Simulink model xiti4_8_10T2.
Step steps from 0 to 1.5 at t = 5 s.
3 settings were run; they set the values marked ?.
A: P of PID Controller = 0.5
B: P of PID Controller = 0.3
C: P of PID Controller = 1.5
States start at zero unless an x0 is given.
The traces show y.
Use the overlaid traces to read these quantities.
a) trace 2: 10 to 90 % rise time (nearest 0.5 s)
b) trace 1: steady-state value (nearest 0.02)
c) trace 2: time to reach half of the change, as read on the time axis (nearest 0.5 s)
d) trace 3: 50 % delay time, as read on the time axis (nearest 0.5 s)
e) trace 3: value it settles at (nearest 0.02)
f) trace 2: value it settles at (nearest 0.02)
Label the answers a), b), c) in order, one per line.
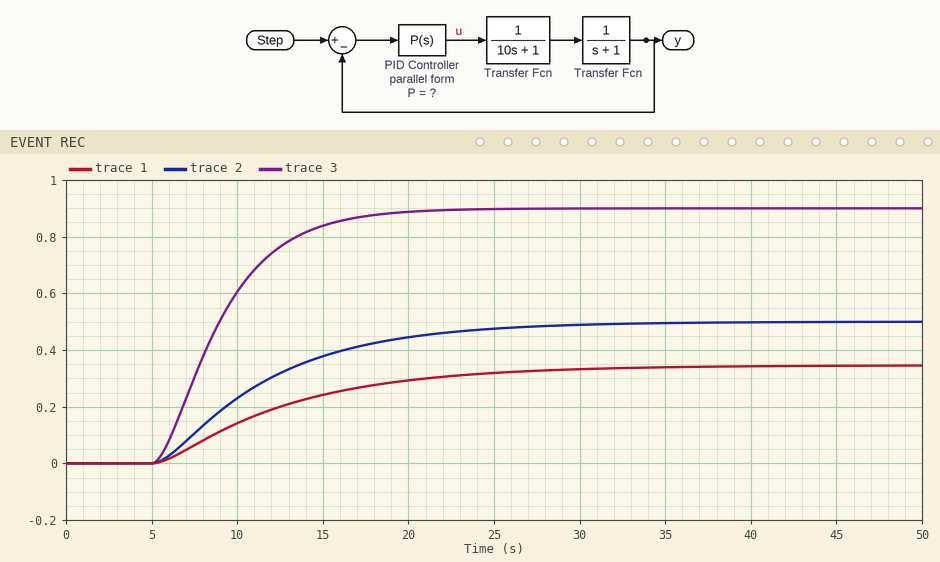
a) 14.0 s
b) 0.34
c) 10.5 s
d) 8.5 s
e) 0.90
f) 0.50
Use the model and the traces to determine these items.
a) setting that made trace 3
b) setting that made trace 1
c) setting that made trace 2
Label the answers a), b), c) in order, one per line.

a) C
b) B
c) A
